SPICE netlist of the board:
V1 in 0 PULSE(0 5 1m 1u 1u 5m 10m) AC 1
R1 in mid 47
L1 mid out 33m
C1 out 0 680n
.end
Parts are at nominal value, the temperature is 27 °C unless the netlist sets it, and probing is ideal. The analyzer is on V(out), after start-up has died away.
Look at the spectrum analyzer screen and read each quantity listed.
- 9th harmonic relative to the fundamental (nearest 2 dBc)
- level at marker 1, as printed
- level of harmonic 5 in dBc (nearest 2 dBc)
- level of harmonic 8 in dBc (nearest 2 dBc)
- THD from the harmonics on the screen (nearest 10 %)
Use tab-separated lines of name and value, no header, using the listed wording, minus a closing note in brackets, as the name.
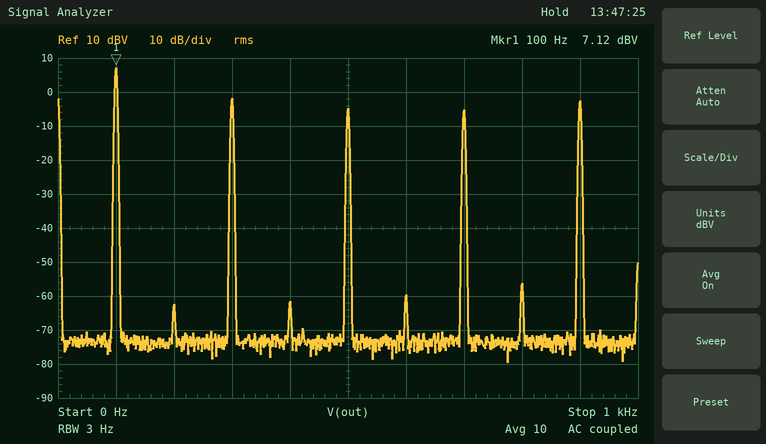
9th harmonic relative to the fundamental	-10 dBc
level at marker 1, as printed	7.12 dBV
level of harmonic 5 in dBc	-12 dBc
level of harmonic 8 in dBc	-64 dBc
THD from the harmonics on the screen	60 %
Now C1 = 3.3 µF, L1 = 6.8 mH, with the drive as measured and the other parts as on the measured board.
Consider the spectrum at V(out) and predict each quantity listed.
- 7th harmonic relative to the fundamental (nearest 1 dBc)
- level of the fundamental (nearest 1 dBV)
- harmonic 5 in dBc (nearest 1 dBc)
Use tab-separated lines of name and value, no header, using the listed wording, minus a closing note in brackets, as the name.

7th harmonic relative to the fundamental	-16 dBc
level of the fundamental	7 dBV
harmonic 5 in dBc	-13 dBc
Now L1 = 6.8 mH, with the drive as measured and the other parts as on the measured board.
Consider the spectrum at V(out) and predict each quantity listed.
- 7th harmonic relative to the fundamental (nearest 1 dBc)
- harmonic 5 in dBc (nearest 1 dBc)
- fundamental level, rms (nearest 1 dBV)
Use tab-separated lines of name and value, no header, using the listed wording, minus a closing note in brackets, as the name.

7th harmonic relative to the fundamental	-16 dBc
harmonic 5 in dBc	-14 dBc
fundamental level, rms	7 dBV
